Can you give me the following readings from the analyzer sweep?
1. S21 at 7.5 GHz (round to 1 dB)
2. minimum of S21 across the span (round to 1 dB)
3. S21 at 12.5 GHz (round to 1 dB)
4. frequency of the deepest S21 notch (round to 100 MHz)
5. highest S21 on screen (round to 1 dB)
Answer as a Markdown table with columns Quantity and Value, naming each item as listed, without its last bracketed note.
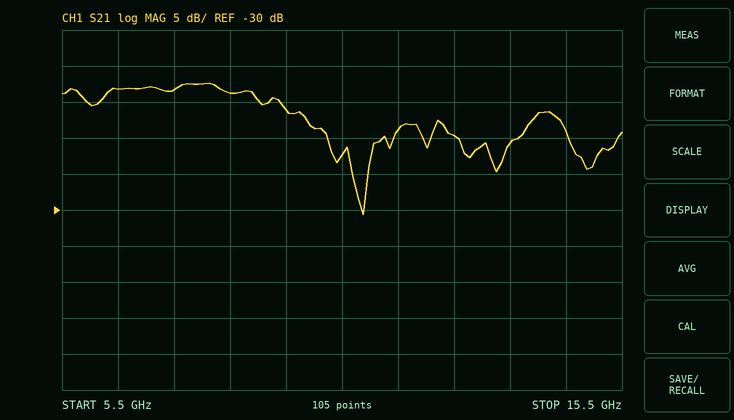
| Quantity | Value |
|---|---|
| S21 at 7.5 GHz | -13 dB |
| minimum of S21 across the span | -31 dB |
| S21 at 12.5 GHz | -20 dB |
| frequency of the deepest S21 notch | 10.9 GHz |
| highest S21 on screen | -12 dB |
